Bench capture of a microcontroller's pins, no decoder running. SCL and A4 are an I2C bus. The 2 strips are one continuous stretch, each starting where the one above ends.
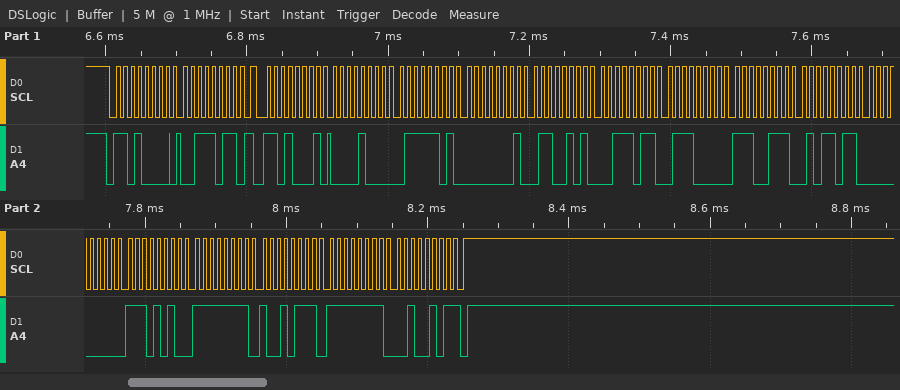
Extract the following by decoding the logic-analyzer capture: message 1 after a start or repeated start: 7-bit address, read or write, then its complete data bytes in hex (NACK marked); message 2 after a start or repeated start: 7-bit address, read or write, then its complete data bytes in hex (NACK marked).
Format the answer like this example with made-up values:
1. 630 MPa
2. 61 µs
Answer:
1. 0x68 write: 3B
2. 0x68 read: 08 7D 01 65 3B 70 E7 5B 00 EA FF 97 FF 25 NACK
